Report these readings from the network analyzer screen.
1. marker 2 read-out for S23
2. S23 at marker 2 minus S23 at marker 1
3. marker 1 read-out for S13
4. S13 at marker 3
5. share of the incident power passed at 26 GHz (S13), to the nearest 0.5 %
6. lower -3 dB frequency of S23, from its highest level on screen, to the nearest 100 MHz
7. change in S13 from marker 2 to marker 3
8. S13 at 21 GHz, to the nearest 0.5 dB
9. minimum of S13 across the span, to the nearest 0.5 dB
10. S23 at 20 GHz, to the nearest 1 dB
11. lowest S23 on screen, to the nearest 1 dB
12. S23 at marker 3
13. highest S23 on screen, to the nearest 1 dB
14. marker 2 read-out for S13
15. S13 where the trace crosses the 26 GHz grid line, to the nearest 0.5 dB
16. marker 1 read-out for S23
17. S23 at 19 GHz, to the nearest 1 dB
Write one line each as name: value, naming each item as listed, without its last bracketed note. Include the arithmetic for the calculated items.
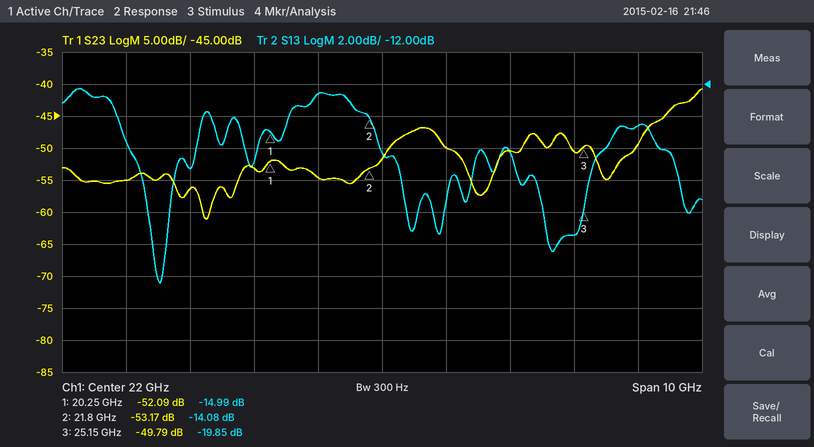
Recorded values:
marker 2 read-out for S23: -53.17 dB
S23 at marker 2 minus S23 at marker 1: -53.17 − (-52.09) = -1.08 dB
marker 1 read-out for S13: -14.99 dB
S13 at marker 3: -19.85 dB
share of the incident power passed at 26 GHz (S13), to the nearest 0.5 %: 10^(-14.5/10) ≈ 3.5 %
lower -3 dB frequency of S23, from its highest level on screen, to the nearest 100 MHz: 26.5 GHz
change in S13 from marker 2 to marker 3: -19.85 − (-14.08) = -5.77 dB
S13 at 21 GHz, to the nearest 0.5 dB: -12.5 dB
minimum of S13 across the span, to the nearest 0.5 dB: -24.5 dB
S23 at 20 GHz, to the nearest 1 dB: -53 dB
lowest S23 on screen, to the nearest 1 dB: -61 dB
S23 at marker 3: -49.79 dB
highest S23 on screen, to the nearest 1 dB: -41 dB
marker 2 read-out for S13: -14.08 dB
S13 where the trace crosses the 26 GHz grid line, to the nearest 0.5 dB: -14.5 dB
marker 1 read-out for S23: -52.09 dB
S23 at 19 GHz, to the nearest 1 dB: -56 dB
